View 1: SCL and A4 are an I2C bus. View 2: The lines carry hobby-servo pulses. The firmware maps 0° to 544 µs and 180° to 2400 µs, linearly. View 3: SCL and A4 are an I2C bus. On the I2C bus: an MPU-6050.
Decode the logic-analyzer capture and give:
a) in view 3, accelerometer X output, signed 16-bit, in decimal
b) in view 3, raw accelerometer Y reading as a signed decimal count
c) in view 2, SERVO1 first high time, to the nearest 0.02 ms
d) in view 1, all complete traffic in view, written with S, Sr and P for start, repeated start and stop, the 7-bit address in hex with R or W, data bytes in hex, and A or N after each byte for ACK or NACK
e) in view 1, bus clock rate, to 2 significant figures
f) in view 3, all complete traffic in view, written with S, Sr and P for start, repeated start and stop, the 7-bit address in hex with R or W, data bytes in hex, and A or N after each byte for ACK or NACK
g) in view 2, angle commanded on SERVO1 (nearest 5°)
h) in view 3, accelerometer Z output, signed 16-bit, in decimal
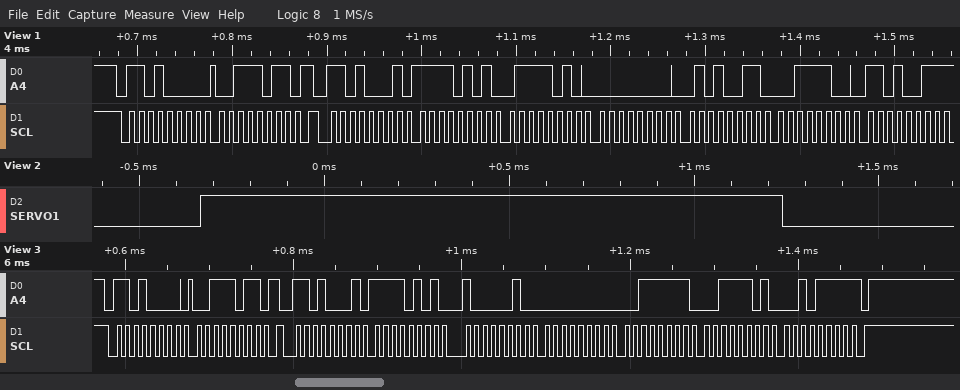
-2686
63
1.58 ms
S 68W A 3B A Sr 68R A F5 A 7A A 00 A 53 A 3C A D3 N
100 kHz
S 68W A 3B A Sr 68R A F5 A 82 A 00 A 3F A 3D A 2F N P
100°
15663
